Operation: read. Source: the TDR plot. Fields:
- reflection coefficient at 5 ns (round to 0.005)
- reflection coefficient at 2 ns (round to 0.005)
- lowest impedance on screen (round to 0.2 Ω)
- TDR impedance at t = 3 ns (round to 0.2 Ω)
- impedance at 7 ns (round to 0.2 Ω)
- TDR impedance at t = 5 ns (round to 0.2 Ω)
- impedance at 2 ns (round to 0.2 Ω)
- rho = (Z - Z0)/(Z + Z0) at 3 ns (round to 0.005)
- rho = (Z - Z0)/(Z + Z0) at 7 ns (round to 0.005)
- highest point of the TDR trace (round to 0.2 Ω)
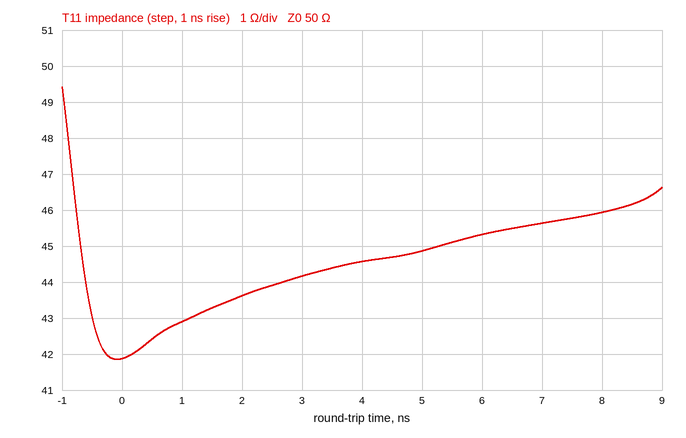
-0.055
-0.070
41.8 Ω
44.2 Ω
45.6 Ω
44.8 Ω
43.6 Ω
-0.060
-0.045
49.4 Ω
